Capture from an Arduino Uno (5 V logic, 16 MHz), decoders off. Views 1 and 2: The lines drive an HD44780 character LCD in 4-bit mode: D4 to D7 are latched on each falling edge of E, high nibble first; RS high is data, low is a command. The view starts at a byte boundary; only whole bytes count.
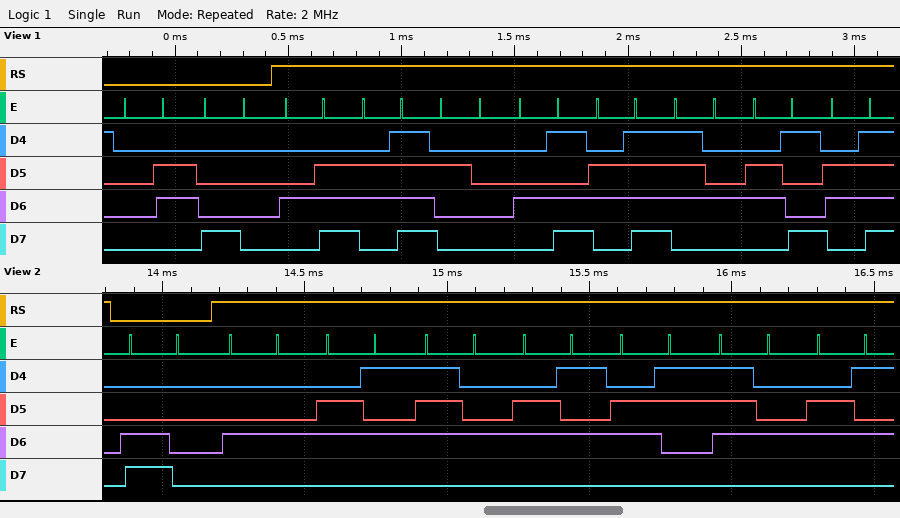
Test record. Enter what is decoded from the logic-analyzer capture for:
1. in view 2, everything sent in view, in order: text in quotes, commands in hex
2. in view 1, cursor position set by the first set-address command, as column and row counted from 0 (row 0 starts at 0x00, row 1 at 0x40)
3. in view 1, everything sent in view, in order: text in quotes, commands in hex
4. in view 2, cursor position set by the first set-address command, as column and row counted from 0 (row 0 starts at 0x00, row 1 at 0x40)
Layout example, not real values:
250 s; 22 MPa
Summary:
0xC0 "Detecte"; column 0, row 0; 0x06 0x80 "No Motio"; column 0, row 1
